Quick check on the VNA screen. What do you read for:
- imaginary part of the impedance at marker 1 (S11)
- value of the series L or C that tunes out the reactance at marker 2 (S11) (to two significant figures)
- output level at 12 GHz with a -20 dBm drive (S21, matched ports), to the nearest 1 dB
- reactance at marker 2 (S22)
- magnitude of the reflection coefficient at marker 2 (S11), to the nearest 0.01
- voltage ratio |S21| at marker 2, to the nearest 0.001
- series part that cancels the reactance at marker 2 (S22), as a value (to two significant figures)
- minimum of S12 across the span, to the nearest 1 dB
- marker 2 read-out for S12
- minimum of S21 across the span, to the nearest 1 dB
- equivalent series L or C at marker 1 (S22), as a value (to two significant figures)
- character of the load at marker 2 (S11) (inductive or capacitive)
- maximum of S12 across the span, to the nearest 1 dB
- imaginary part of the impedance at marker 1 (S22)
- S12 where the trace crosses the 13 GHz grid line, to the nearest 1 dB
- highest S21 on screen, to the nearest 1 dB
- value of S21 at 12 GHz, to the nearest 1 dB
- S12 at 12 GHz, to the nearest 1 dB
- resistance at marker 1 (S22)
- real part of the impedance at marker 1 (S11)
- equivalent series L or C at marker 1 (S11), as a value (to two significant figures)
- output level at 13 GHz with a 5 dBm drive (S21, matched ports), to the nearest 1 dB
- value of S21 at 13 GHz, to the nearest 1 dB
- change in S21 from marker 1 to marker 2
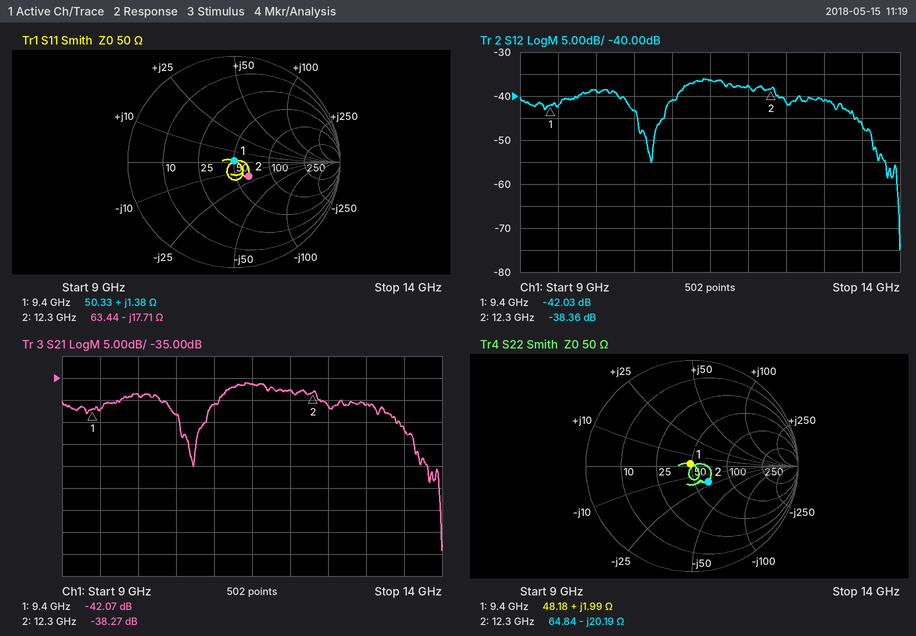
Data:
+1.38 Ω
230 pH
-58 dBm
-20.19 Ω
0.19
0.012
260 pH
-75 dB
-38.36 dB
-74 dB
34 pH
capacitive
-36 dB
+1.99 Ω
-41 dB
-36 dB
-38 dB
-38 dB
48.18 Ω
50.33 Ω
23 pH
-36 dBm
-41 dB
3.80 dB
